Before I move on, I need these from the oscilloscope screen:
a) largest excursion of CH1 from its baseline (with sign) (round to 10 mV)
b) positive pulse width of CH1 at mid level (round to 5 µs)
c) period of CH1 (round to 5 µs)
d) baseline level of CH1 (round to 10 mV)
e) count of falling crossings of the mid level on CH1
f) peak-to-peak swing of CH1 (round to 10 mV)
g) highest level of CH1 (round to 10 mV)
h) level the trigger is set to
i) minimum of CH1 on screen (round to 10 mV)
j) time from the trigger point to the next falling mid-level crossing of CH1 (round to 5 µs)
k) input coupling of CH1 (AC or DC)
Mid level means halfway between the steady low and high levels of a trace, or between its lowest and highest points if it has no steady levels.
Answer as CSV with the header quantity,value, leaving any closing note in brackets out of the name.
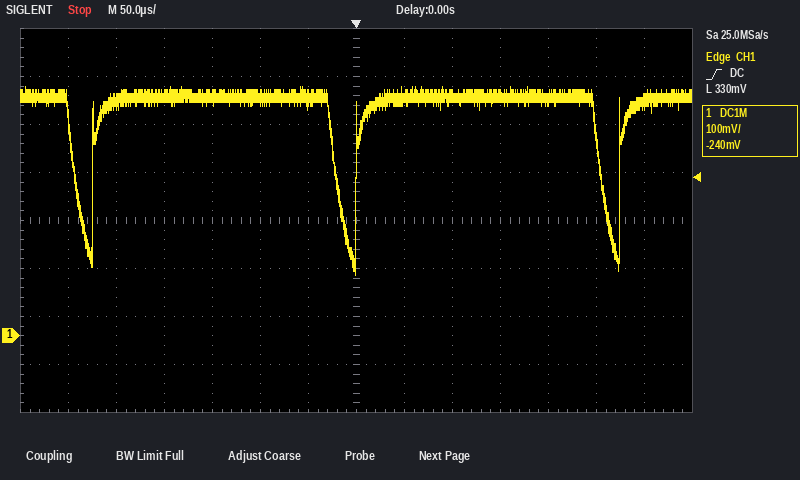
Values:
quantity,value
largest excursion of CH1 from its baseline (with sign),-370 mV
positive pulse width of CH1 at mid level,255 µs
period of CH1,275 µs
baseline level of CH1,500 mV
count of falling crossings of the mid level on CH1,3
peak-to-peak swing of CH1,390 mV
highest level of CH1,520 mV
level the trigger is set to,330 mV
minimum of CH1 on screen,130 mV
time from the trigger point to the next falling mid-level crossing of CH1,255 µs
input coupling of CH1,DC
